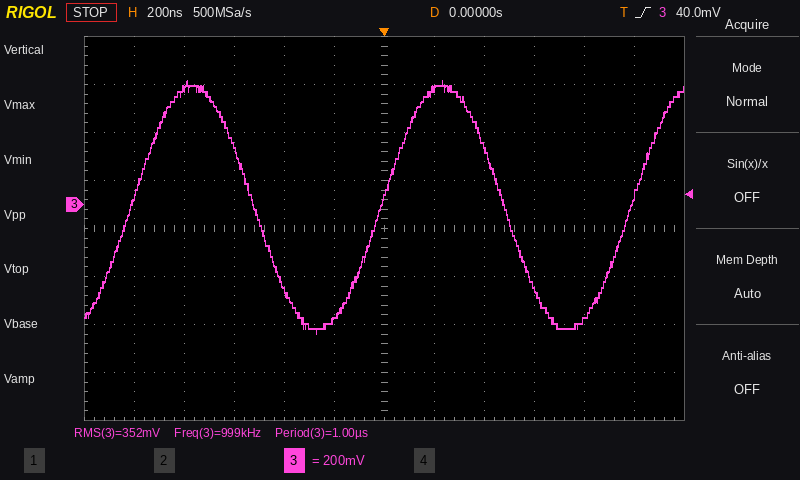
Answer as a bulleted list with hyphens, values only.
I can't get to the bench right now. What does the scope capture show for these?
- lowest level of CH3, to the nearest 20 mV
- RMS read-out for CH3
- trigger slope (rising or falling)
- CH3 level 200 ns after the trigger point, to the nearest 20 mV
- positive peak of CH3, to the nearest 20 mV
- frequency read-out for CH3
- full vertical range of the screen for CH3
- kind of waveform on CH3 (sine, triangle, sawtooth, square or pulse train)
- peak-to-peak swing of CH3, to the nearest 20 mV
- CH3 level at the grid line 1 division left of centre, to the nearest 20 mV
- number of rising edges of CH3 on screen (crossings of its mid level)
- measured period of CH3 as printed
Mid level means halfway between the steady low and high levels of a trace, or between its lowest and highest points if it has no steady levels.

- -540 mV
- 352 mV
- rising
- 480 mV
- 520 mV
- 999 kHz
- 1.6 V
- sine
- 1.06 V
- -480 mV
- 3
- 1.00 µs
